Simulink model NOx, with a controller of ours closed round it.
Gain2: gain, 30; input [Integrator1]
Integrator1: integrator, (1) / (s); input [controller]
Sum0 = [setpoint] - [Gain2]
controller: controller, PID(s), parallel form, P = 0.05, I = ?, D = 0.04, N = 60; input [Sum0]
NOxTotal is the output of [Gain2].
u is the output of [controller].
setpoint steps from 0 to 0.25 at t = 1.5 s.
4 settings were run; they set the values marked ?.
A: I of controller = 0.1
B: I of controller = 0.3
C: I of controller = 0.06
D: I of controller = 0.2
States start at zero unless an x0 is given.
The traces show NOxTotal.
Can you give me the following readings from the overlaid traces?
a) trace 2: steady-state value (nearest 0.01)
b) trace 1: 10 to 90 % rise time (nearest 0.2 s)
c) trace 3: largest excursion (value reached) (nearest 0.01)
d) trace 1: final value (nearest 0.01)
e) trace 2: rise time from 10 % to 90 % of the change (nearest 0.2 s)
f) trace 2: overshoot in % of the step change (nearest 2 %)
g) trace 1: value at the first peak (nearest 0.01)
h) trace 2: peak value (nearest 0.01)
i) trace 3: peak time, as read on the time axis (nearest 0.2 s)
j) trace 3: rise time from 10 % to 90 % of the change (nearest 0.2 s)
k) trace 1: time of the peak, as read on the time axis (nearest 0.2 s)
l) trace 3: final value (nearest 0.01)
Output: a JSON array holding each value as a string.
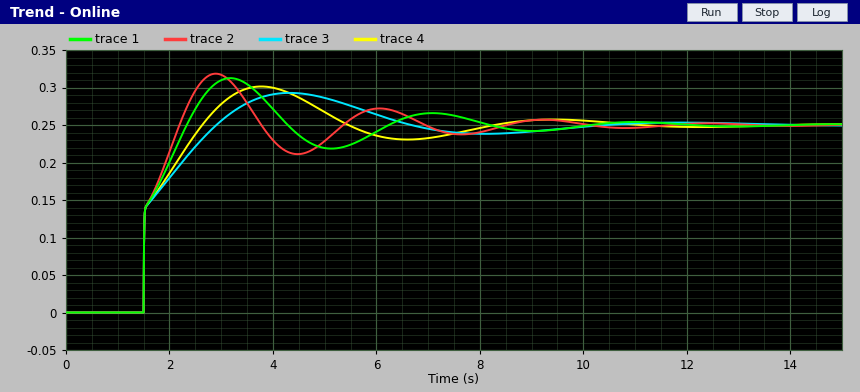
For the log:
["0.25", "0.6 s", "0.29", "0.25", "0.6 s", "28 %", "0.31", "0.32", "4.4 s", "1.0 s", "3.2 s", "0.25"]
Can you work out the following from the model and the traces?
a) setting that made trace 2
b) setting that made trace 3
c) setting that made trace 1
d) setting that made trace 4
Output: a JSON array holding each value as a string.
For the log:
["B", "C", "D", "A"]
